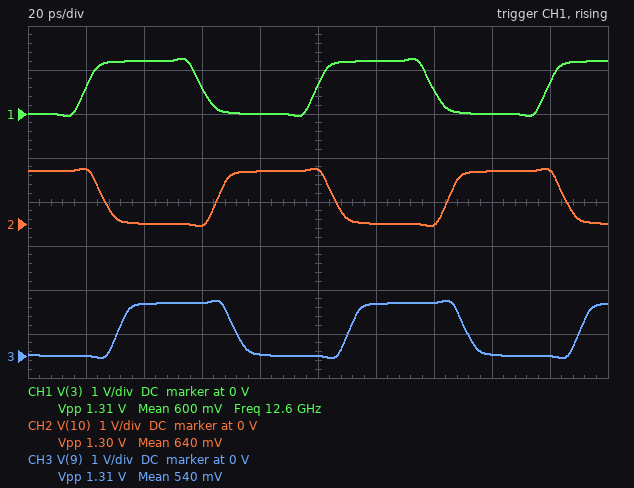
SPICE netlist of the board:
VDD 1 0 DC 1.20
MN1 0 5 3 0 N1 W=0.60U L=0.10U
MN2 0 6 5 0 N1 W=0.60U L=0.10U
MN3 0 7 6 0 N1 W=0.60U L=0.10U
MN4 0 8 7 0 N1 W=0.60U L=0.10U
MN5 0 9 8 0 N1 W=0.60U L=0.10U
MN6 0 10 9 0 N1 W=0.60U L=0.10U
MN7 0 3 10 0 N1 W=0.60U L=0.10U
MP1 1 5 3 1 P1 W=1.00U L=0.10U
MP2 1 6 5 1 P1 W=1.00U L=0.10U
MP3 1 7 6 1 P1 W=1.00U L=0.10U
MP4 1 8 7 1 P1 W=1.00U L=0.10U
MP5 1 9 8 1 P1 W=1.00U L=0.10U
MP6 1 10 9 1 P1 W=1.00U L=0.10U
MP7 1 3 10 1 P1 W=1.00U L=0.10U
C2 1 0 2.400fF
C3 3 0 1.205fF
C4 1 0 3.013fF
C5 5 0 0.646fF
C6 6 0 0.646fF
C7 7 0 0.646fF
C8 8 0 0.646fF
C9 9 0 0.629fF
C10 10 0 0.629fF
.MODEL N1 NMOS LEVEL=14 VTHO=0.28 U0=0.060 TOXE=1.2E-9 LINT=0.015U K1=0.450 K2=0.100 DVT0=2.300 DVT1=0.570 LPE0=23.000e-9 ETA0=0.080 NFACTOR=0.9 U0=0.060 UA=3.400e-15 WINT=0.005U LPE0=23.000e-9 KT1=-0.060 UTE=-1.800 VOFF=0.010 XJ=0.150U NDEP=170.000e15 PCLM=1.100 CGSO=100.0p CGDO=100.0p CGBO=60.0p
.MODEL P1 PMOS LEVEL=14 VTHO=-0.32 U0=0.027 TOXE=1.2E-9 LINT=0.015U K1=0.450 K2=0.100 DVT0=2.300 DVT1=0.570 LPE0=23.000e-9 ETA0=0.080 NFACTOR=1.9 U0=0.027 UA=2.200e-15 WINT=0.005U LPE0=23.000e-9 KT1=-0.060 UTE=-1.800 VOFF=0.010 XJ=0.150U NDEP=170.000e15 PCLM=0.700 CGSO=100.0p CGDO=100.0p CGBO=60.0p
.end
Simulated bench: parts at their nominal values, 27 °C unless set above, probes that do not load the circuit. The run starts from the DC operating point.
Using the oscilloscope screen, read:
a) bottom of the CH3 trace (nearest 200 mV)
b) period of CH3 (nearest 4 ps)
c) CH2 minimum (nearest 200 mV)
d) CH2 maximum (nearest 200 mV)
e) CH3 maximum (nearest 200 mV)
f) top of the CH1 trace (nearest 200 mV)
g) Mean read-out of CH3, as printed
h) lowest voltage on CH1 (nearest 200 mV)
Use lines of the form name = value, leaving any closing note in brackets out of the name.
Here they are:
bottom of the CH3 trace = 0 V
period of CH3 = 80 ps
CH2 minimum = 0 V
CH2 maximum = 1.2 V
CH3 maximum = 1.2 V
top of the CH1 trace = 1.2 V
Mean read-out of CH3, as printed = 540 mV
lowest voltage on CH1 = 0 V
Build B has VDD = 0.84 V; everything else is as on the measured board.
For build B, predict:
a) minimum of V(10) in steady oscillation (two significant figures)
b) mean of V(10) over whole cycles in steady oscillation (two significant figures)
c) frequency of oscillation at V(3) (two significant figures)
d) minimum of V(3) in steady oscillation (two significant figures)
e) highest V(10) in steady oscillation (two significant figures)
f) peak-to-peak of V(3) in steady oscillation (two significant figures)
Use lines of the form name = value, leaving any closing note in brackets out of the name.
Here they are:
minimum of V(10) in steady oscillation = -64 mV
mean of V(10) over whole cycles in steady oscillation = 420 mV
frequency of oscillation at V(3) = 8.1 GHz
minimum of V(3) in steady oscillation = -63 mV
highest V(10) in steady oscillation = 920 mV
peak-to-peak of V(3) in steady oscillation = 980 mV
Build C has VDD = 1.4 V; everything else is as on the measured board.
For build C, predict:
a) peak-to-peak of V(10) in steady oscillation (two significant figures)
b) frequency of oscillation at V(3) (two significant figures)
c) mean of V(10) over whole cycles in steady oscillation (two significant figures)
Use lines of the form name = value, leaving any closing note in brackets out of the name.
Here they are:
peak-to-peak of V(10) in steady oscillation = 1.5 V
frequency of oscillation at V(3) = 14 GHz
mean of V(10) over whole cycles in steady oscillation = 710 mV
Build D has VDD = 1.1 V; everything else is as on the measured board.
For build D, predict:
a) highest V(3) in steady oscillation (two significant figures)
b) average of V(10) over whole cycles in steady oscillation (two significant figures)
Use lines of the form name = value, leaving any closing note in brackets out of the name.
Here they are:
highest V(3) in steady oscillation = 1.2 V
average of V(10) over whole cycles in steady oscillation = 550 mV
